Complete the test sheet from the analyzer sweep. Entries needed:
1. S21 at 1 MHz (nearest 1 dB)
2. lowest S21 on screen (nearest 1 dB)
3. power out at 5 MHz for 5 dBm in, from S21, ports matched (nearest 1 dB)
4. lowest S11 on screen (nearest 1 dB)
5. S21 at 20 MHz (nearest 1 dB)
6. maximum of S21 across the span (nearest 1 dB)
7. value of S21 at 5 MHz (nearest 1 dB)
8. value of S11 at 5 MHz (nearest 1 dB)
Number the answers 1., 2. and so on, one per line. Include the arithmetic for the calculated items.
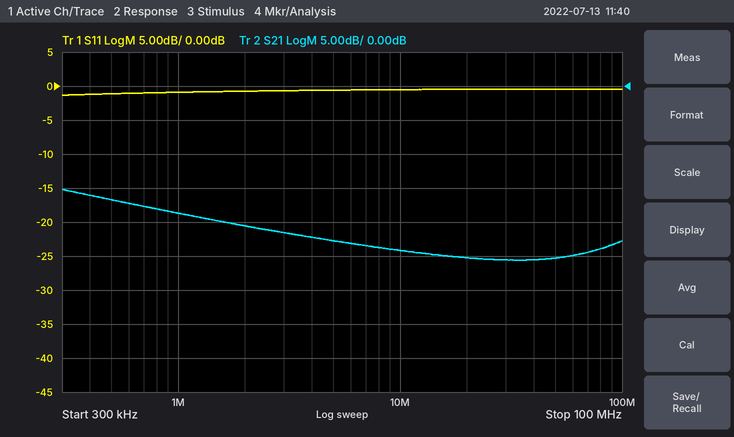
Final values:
1. -19 dB
2. -26 dB
3. 5 dBm + (-23 dB) = -18 dBm
4. -1 dB
5. -25 dB
6. -15 dB
7. -23 dB
8. -1 dB
